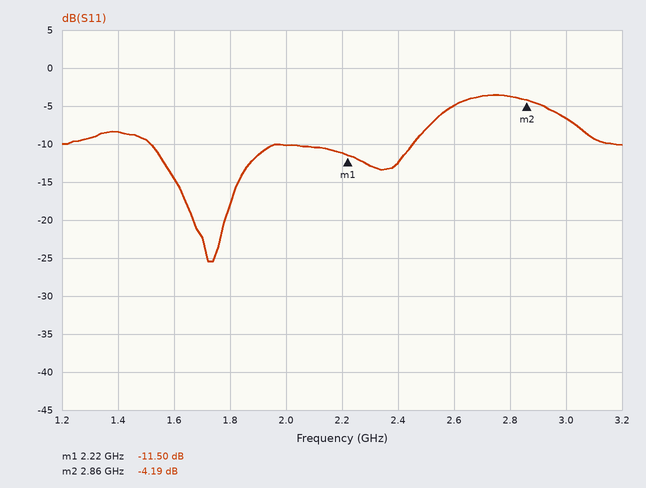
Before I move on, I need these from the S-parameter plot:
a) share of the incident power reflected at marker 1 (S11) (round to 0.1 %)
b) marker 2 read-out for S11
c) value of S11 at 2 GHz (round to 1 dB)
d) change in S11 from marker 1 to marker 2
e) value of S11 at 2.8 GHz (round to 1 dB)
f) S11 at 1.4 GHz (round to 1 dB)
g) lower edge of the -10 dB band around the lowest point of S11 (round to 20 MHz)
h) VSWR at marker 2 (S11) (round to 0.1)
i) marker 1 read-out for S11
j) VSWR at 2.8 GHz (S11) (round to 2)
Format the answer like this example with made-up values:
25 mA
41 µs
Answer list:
7.1 %
-4.19 dB
-10 dB
7.31 dB
-4 dB
-8 dB
1.52 GHz
4.2
-11.50 dB
4
